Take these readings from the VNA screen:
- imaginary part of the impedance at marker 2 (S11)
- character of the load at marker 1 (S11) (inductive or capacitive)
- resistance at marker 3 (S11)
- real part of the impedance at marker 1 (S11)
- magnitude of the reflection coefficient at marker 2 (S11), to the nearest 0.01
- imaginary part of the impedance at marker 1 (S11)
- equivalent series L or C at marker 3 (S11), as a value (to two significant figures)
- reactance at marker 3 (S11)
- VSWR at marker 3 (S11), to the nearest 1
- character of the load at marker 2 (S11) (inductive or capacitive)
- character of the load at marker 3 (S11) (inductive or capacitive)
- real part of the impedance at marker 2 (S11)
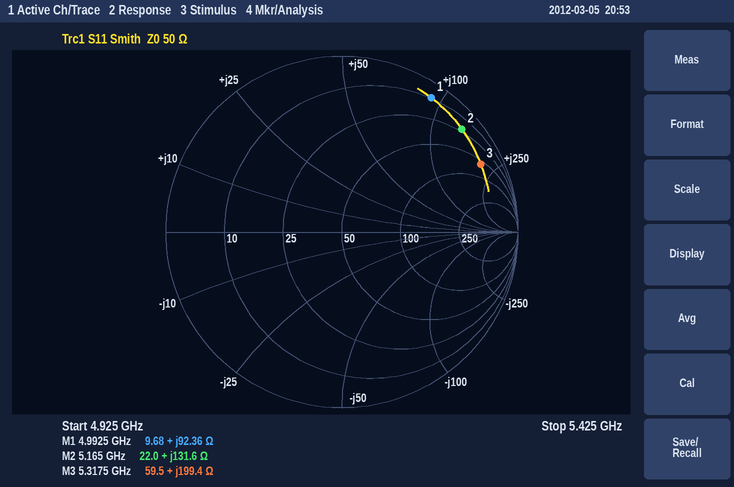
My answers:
+131.6 Ω
inductive
59.5 Ω
9.68 Ω
0.90
+92.36 Ω
6.0 nH
+199.4 Ω
15
inductive
inductive
22.0 Ω
